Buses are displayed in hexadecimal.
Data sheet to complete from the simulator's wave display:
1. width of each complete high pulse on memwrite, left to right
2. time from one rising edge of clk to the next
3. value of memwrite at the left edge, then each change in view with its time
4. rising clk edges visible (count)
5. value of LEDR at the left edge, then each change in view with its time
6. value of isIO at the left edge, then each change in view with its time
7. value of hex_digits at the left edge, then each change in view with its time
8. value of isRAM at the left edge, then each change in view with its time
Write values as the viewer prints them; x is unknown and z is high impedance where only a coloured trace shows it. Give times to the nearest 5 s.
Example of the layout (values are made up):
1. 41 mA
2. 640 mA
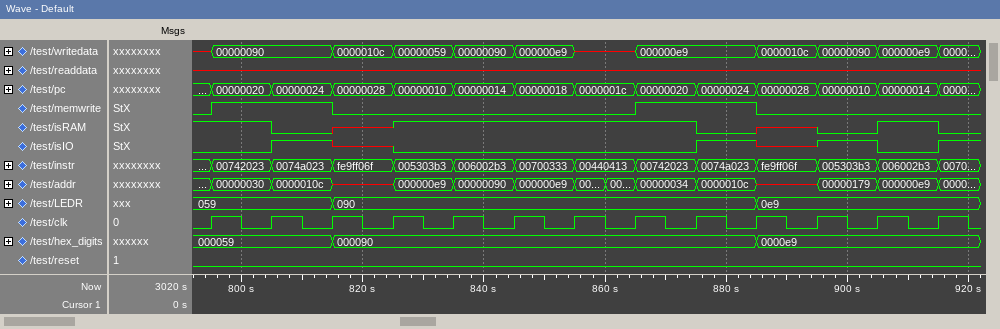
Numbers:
1. 20 s, 20 s
2. 10 s
3. 0, 1 at 795 s, 0 at 815 s, 1 at 865 s, 0 at 885 s
4. 13
5. 059, 090 at 815 s, 0e9 at 885 s
6. 0, 1 at 805 s, x at 815 s, 0 at 825 s, 1 at 875 s, x at 885 s, 1 at 895 s, 0 at 905 s, 1 at 915 s
7. 000059, 000090 at 815 s, 0000e9 at 885 s
8. 1, 0 at 805 s, x at 815 s, 1 at 825 s, 0 at 875 s, x at 885 s, 0 at 895 s, 1 at 905 s, 0 at 915 s
